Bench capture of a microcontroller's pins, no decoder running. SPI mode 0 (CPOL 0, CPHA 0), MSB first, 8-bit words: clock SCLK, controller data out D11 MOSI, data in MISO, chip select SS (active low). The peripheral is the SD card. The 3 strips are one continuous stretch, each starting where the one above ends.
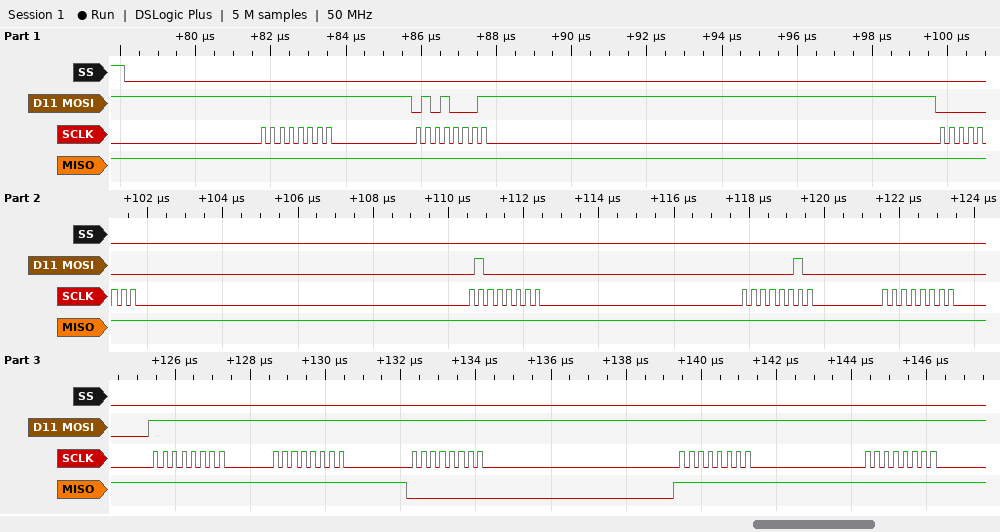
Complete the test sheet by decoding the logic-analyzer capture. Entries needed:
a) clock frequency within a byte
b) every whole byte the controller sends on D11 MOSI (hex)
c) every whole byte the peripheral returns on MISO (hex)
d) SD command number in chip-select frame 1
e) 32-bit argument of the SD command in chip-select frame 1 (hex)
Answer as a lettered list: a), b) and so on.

a) 4 MHz
b) FF 51 00 40 02 00 FF FF FF FF FF
c) FF FF FF FF FF FF FF FF 00 FF FF
d) CMD17
e) 0x00400200
